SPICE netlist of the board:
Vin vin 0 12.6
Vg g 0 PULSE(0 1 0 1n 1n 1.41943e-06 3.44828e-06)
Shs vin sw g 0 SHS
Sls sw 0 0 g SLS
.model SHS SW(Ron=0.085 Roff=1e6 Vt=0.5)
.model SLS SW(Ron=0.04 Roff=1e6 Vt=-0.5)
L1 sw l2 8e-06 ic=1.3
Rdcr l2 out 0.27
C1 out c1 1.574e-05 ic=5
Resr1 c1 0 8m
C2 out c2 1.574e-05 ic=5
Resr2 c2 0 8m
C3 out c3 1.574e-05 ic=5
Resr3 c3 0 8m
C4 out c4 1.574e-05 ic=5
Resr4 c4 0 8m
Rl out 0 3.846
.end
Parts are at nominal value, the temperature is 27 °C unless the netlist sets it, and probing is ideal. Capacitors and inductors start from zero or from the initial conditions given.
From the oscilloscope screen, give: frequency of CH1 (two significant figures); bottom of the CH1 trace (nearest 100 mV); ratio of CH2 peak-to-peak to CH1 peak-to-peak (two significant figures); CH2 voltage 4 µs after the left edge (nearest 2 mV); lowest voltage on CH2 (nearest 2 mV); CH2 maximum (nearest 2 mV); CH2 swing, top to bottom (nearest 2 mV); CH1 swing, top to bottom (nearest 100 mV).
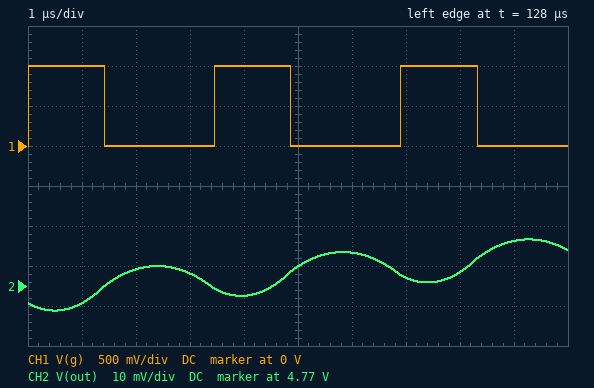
290 kHz
0 V
0.018
4.768 V
4.764 V
4.782 V
18 mV
1.0 V
